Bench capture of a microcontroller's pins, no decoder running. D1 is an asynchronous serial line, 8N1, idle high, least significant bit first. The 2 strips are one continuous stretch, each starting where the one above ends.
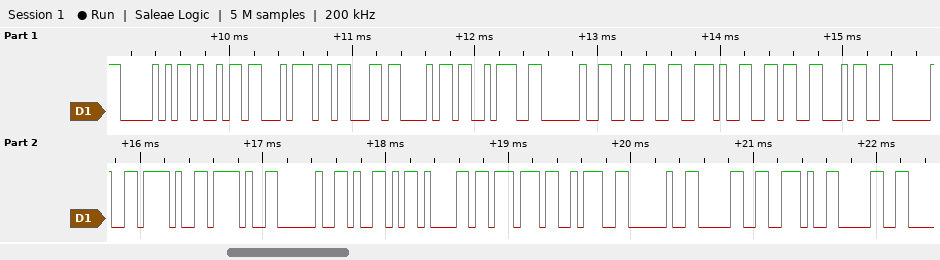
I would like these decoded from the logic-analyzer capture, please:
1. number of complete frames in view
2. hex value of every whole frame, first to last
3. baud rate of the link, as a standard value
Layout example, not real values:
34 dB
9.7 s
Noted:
23
50 69 74 63 68 3A 20 32 2E 36 34 20 2F 2F 20 59 61 77 3A 20 30 2E 30
19200 baud
